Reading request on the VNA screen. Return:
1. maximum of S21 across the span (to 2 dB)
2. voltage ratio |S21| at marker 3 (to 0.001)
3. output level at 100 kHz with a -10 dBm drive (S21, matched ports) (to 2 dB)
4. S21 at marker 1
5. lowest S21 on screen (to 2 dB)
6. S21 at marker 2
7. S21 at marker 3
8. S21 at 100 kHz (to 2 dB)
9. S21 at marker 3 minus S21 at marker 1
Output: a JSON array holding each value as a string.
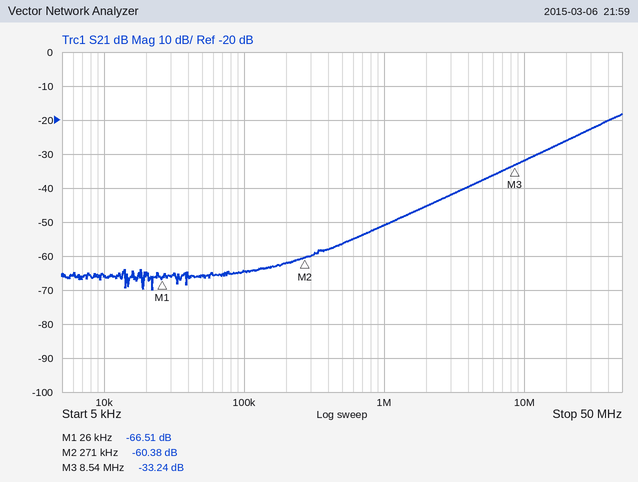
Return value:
["-18 dB", "0.022", "-74 dBm", "-66.51 dB", "-70 dB", "-60.38 dB", "-33.24 dB", "-64 dB", "33.27 dB"]
